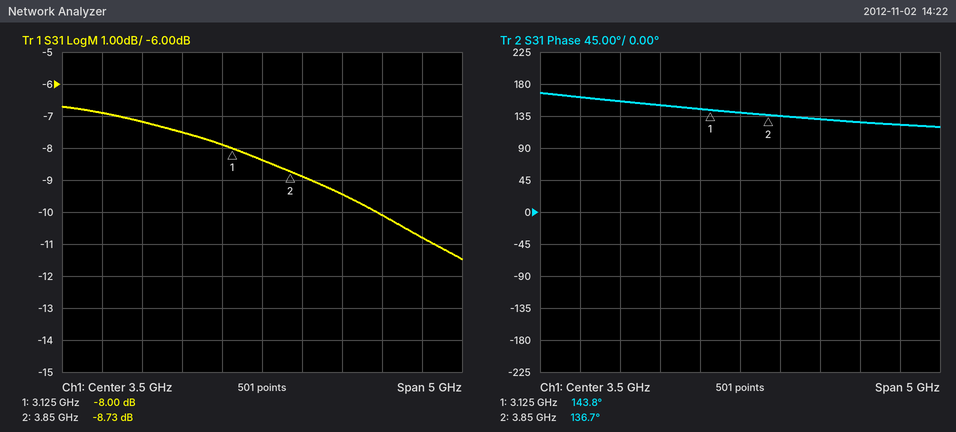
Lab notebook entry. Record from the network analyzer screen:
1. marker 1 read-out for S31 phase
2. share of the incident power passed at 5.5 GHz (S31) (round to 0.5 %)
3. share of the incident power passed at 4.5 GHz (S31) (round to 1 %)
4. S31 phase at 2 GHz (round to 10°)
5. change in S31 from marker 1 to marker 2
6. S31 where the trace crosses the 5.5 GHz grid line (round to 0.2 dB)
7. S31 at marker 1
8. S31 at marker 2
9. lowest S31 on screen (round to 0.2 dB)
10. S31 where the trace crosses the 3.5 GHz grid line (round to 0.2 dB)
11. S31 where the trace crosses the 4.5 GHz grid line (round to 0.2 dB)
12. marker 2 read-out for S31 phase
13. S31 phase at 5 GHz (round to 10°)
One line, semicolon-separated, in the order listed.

143.8°; 8.5 %; 11 %; 160°; -0.73 dB; -10.8 dB; -8.00 dB; -8.73 dB; -11.4 dB; -8.4 dB; -9.4 dB; 136.7°; 130°
